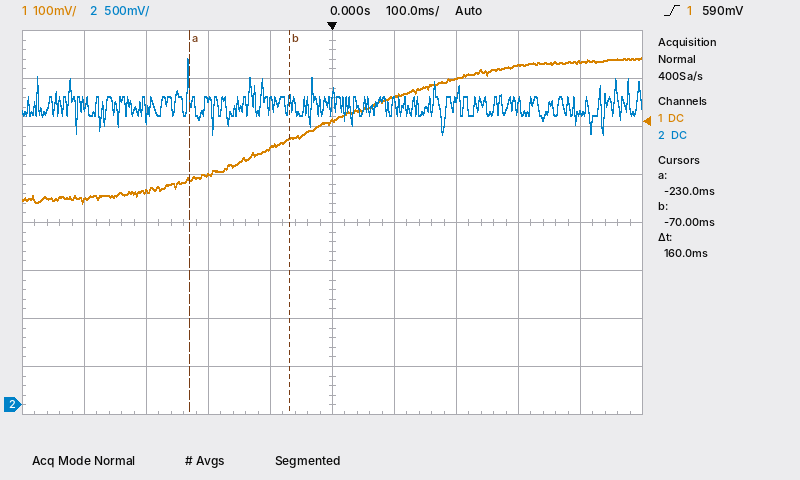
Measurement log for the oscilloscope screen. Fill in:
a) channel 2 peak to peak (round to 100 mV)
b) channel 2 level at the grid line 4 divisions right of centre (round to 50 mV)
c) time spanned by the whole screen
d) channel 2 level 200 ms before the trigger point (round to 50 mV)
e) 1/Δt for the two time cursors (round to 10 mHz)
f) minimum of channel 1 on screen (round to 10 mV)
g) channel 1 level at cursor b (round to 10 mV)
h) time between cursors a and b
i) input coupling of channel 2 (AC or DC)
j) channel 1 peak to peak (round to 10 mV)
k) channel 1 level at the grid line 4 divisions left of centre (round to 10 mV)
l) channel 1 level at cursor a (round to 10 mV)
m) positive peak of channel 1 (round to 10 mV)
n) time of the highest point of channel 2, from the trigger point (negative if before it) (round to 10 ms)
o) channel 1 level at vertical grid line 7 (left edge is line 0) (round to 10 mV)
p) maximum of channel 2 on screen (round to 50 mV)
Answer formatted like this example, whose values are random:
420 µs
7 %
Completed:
800 mV
3.05 V
1 s
3.20 V
6.25 Hz
420 mV
550 mV
160 ms
DC
300 mV
430 mV
470 mV
720 mV
-230 ms
680 mV
3.60 V
